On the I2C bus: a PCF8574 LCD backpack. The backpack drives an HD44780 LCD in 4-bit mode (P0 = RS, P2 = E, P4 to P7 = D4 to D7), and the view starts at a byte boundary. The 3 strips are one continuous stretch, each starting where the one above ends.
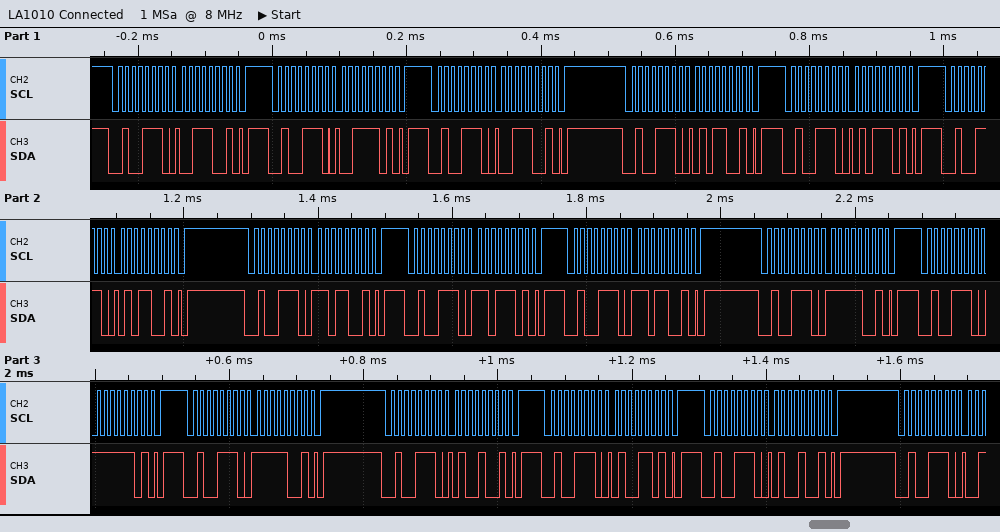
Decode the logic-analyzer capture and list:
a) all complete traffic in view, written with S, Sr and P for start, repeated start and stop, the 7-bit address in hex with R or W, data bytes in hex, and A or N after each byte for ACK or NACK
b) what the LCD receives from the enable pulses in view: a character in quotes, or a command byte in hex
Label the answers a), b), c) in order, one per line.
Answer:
a) S 27W A 39 A P S 27W A 3D A P S 27W A 39 A P S 27W A 59 A P S 27W A 5D A P S 27W A 59 A P S 27W A D9 A P S 27W A DD A P S 27W A D9 A P S 27W A F9 A P S 27W A FD A P S 27W A F9 A P S 27W A 49 A P S 27W A 4D A P S 27W A 49 A P S 27W A
b) '5' data 0xDF
